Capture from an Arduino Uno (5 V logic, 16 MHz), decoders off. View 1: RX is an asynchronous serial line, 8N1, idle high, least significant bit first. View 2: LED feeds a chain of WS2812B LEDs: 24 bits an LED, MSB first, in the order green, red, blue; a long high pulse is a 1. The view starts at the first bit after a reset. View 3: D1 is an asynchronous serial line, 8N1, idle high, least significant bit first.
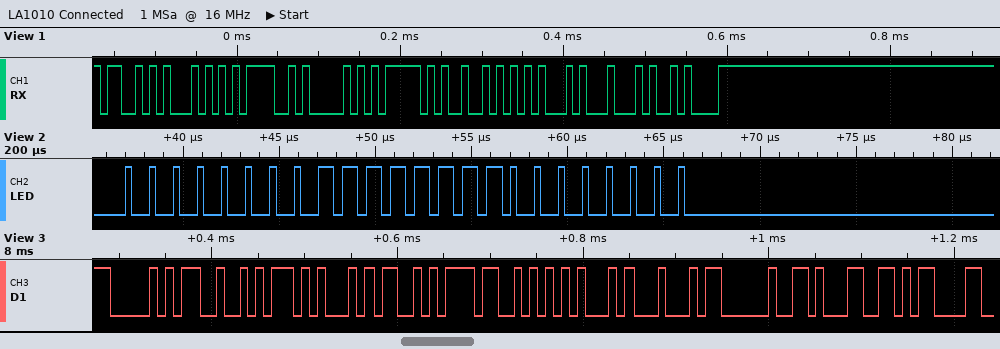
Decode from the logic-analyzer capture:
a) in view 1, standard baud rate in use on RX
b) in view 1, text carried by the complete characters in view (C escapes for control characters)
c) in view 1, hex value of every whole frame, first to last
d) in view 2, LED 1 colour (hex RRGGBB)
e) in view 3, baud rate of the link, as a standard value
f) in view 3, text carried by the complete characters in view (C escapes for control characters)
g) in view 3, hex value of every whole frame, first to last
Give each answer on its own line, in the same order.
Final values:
115200 baud
"STOP_RED\n"
53 54 4F 50 5F 52 45 44 0A
#FF0000
115200 baud
"PRESSED 1\r"
0x50 0x52 0x45 0x53 0x53 0x45 0x44 0x20 0x31 0x0D
